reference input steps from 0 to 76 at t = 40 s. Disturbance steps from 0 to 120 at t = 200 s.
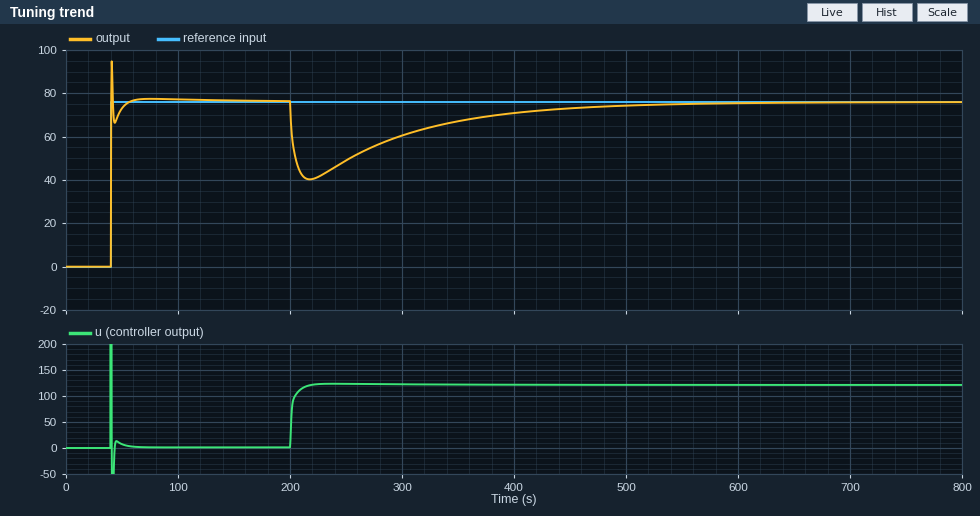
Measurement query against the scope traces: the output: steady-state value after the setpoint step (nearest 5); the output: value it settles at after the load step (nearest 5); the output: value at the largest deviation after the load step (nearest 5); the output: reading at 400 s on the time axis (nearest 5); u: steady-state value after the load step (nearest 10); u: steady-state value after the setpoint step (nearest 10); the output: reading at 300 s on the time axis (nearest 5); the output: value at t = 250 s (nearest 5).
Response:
75
75
40
70
120
0
60
50
